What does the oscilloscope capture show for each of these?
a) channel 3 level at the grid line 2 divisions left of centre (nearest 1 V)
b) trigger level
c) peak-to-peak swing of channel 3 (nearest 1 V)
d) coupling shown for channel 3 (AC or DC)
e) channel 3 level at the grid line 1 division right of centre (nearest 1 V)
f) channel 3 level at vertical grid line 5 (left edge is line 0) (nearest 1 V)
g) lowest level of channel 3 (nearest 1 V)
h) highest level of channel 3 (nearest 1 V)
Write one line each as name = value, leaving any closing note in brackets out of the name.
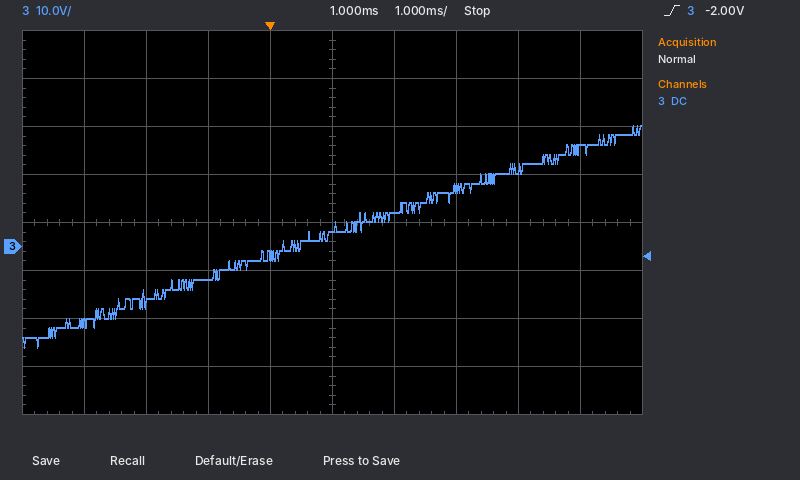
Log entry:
channel 3 level at the grid line 2 divisions left of centre = -7 V
trigger level = -2.00 V
peak-to-peak swing of channel 3 = 46 V
coupling shown for channel 3 = DC
channel 3 level at the grid line 1 division right of centre = 7 V
channel 3 level at vertical grid line 5 (left edge is line 0) = 4 V
lowest level of channel 3 = -21 V
highest level of channel 3 = 25 V
